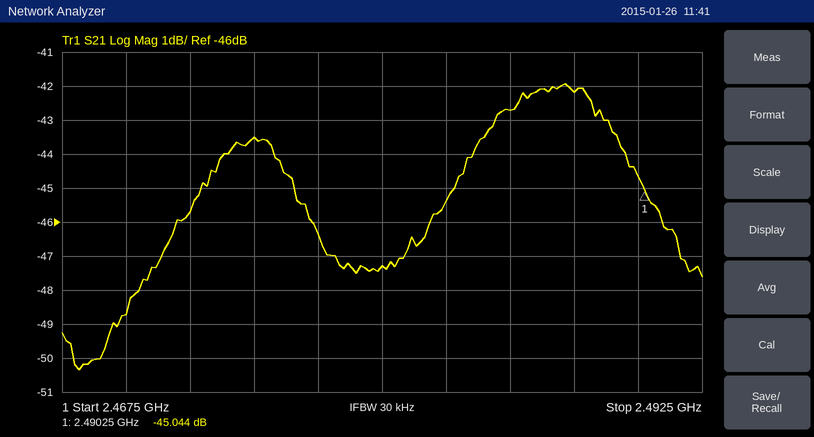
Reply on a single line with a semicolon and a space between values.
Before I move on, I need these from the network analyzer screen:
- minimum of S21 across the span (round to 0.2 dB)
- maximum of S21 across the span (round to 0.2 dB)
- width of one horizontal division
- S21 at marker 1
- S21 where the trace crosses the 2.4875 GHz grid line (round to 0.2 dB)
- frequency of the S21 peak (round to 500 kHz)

-50.4 dB; -42.0 dB; 2.5 MHz; -45.044 dB; -42.2 dB; 2.4870 GHz
